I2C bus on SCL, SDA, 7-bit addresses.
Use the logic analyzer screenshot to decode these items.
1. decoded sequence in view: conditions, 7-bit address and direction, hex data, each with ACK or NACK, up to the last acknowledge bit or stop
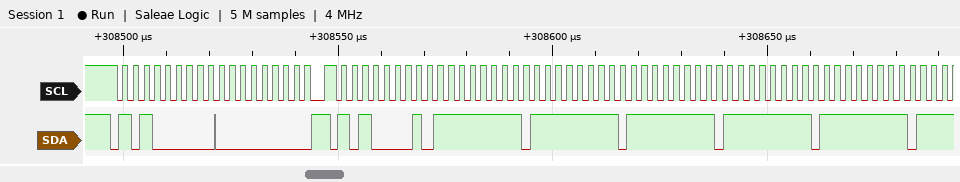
start, address 50 write ACK, 00 ACK, repeated start, address 50 read ACK, FF ACK, FF ACK, FF ACK, FF ACK, FF ACK
